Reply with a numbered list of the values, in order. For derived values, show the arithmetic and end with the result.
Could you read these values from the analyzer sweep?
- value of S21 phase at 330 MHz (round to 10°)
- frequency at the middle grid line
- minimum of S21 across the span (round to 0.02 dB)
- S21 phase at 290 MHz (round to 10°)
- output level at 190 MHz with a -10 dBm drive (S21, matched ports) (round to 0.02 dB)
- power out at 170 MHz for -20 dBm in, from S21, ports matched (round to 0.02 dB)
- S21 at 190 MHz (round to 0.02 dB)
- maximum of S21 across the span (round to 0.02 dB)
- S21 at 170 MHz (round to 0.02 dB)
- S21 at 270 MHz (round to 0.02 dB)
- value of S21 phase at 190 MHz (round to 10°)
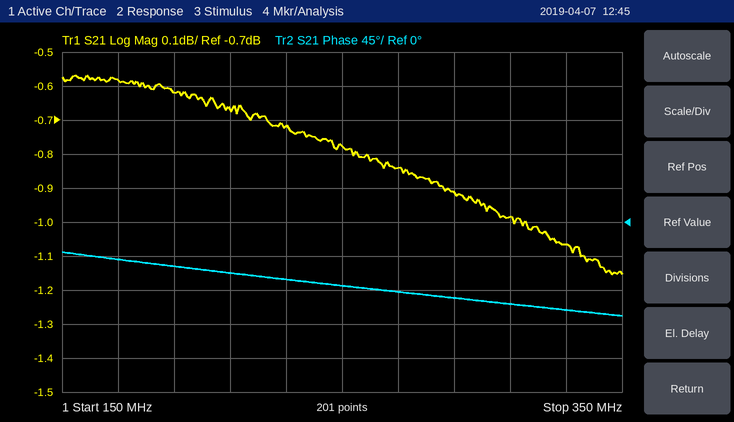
1. -120°
2. 250 MHz
3. -1.16 dB
4. -100°
5. -10 dBm + (-0.62 dB) = -10.62 dBm
6. -20 dBm + (-0.58 dB) = -20.58 dBm
7. -0.62 dB
8. -0.56 dB
9. -0.58 dB
10. -0.84 dB
11. -60°
